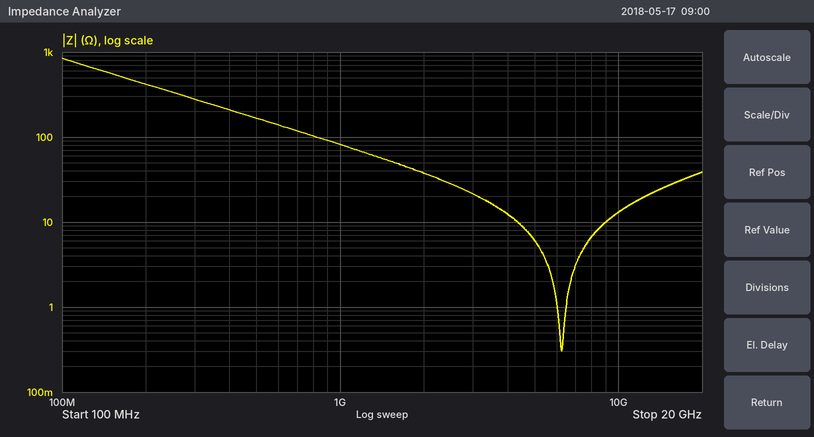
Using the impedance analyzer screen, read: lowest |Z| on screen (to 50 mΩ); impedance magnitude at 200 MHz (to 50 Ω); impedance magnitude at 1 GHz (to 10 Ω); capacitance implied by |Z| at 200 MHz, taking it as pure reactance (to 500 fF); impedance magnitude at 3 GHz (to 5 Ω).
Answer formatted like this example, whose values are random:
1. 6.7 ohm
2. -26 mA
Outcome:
1. 300 mΩ
2. 400 Ω
3. 80 Ω
4. 2.0 pF
5. 20 Ω
